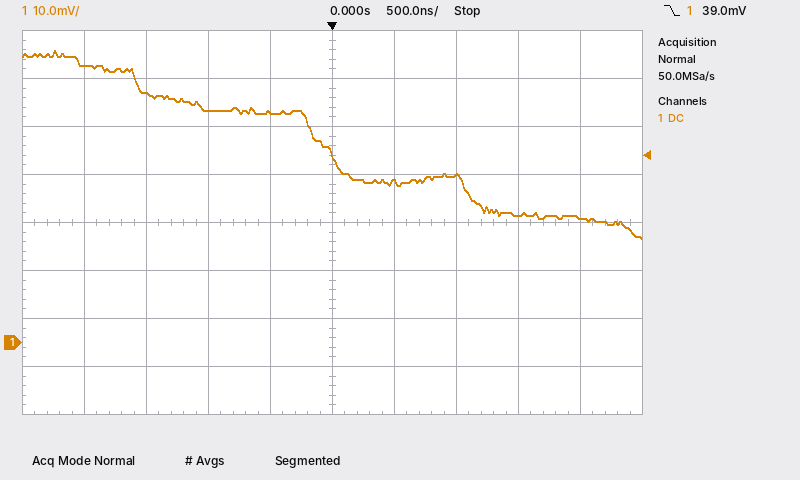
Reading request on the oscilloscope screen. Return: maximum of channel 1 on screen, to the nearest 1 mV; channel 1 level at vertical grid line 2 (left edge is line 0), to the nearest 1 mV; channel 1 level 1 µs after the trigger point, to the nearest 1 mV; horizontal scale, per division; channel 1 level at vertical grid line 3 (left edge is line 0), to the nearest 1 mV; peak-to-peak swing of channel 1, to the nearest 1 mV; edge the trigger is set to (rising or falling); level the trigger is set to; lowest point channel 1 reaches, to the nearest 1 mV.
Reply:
61 mV
52 mV
35 mV
500 ns
48 mV
39 mV
falling
39.0 mV
22 mV
